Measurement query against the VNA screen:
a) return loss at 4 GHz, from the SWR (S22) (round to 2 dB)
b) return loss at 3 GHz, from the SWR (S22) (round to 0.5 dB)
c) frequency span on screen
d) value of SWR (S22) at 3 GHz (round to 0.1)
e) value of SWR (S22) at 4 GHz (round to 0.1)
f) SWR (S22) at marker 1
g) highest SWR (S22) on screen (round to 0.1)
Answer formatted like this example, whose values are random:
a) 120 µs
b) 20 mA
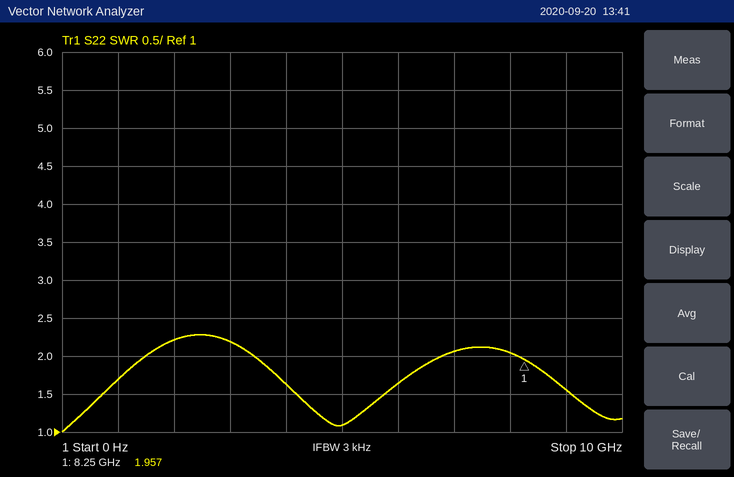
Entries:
a) 12 dB
b) 8.5 dB
c) 10 GHz
d) 2.2
e) 1.6
f) 1.957
g) 2.3
